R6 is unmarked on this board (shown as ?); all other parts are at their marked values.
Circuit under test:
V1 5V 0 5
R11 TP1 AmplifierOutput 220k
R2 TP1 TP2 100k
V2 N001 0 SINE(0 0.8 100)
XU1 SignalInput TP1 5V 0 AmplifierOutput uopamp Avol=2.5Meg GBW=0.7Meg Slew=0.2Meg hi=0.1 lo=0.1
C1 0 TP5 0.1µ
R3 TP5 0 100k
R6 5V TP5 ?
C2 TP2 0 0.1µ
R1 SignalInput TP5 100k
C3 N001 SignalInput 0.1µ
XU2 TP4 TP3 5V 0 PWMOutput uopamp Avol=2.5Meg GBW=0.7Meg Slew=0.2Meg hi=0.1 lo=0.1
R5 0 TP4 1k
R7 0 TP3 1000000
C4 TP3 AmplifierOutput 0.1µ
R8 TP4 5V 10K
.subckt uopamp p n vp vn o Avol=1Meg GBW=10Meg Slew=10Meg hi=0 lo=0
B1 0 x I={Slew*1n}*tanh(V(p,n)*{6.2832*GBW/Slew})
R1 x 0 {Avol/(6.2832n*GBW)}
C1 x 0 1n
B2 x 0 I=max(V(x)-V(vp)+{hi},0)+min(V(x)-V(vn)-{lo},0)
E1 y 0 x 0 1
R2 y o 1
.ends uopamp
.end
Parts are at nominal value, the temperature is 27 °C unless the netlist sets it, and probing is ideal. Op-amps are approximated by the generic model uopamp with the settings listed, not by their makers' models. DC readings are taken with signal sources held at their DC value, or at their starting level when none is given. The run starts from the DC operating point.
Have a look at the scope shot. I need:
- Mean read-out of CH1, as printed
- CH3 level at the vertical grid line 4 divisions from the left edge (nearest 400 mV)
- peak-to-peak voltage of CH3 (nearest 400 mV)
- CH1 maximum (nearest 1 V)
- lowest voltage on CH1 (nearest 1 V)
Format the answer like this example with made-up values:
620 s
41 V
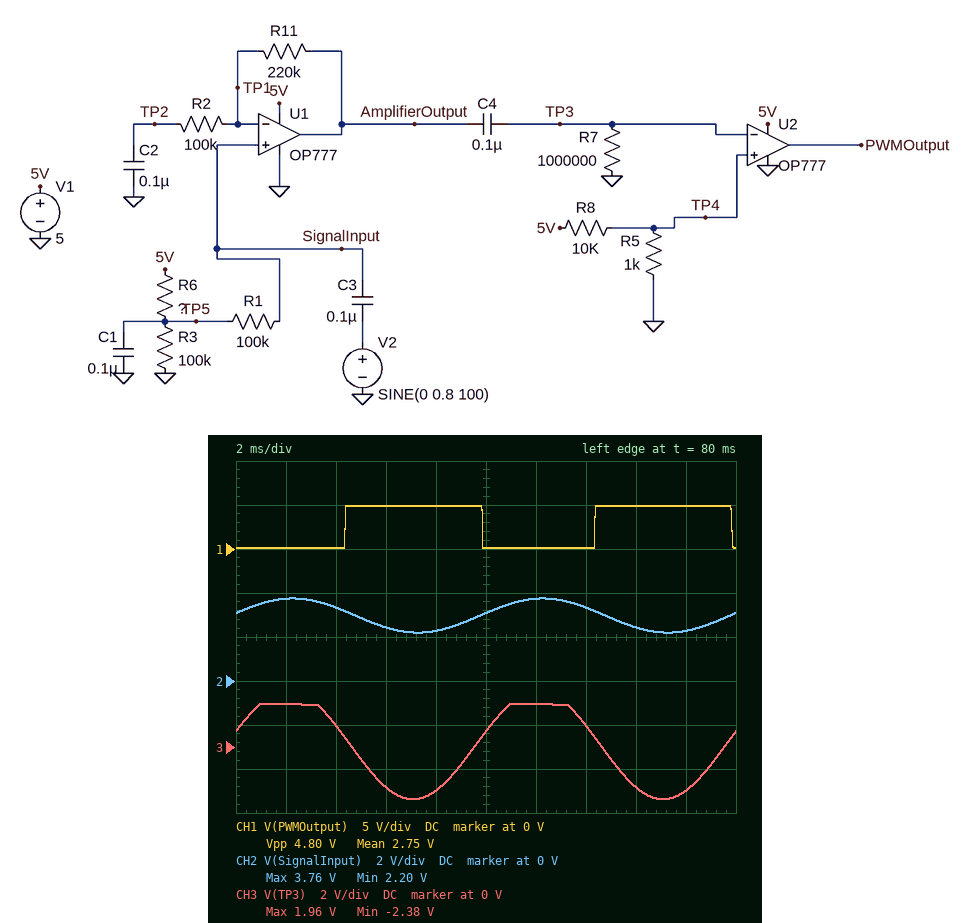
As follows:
2.75 V
-2.0 V
4.4 V
5 V
0 V
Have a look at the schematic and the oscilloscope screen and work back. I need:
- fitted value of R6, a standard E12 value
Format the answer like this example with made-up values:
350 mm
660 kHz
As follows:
68 kΩ
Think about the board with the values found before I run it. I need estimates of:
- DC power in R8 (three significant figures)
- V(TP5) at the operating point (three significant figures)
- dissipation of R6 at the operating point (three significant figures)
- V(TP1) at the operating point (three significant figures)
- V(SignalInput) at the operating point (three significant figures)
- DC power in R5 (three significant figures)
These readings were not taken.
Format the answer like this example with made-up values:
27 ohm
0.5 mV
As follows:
2.07 mW
2.98 V
60.2 µW
2.98 V
2.98 V
207 µW
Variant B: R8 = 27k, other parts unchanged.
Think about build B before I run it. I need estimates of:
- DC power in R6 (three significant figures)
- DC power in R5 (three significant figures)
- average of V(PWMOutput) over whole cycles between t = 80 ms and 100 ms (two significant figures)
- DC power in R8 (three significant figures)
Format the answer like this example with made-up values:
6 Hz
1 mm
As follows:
60.2 µW
31.9 µW
2.6 V
861 µW
